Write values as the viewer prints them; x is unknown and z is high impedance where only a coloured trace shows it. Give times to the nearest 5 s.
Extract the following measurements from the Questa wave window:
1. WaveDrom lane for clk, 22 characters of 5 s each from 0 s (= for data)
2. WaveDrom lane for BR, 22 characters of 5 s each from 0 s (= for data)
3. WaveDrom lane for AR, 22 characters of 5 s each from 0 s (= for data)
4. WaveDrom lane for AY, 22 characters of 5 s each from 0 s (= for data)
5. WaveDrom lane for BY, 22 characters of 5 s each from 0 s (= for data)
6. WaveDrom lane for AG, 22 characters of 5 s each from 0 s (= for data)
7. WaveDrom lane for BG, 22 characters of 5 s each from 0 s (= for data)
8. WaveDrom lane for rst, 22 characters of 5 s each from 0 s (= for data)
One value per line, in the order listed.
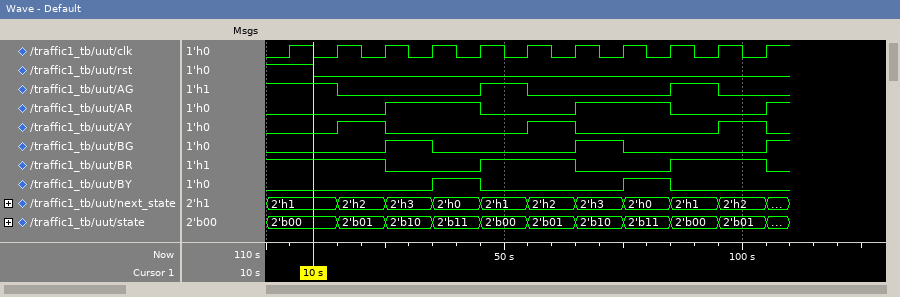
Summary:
{name: 'clk', wave: '0101010101010101010101'}
{name: 'BR', wave: '1....0...1...0...1...0'}
{name: 'AR', wave: '0....1...0...1...0...1'}
{name: 'AY', wave: '0..1.0.....1.0.....1.0'}
{name: 'BY', wave: '0......1.0.....1.0....'}
{name: 'AG', wave: '1..0.....1.0.....1.0..'}
{name: 'BG', wave: '0....1.0.....1.0.....1'}
{name: 'rst', wave: '1.0...................'}
